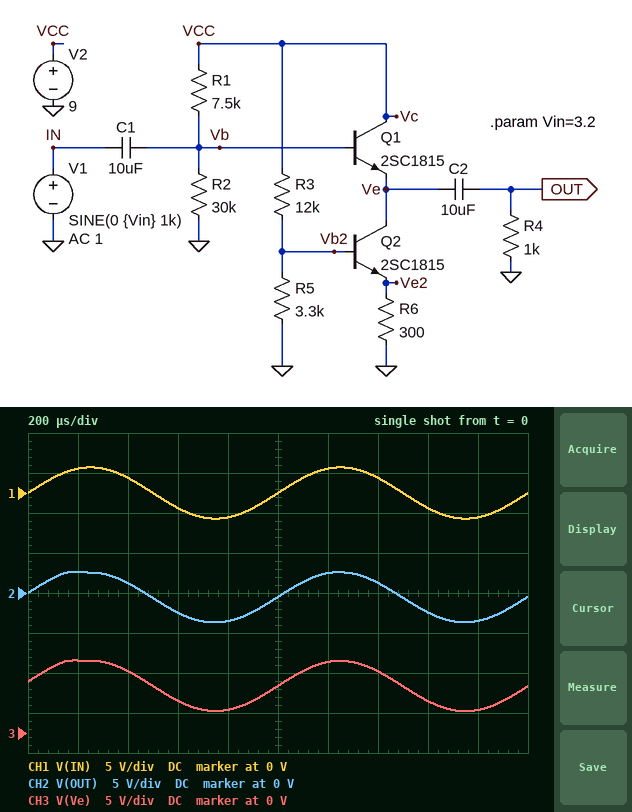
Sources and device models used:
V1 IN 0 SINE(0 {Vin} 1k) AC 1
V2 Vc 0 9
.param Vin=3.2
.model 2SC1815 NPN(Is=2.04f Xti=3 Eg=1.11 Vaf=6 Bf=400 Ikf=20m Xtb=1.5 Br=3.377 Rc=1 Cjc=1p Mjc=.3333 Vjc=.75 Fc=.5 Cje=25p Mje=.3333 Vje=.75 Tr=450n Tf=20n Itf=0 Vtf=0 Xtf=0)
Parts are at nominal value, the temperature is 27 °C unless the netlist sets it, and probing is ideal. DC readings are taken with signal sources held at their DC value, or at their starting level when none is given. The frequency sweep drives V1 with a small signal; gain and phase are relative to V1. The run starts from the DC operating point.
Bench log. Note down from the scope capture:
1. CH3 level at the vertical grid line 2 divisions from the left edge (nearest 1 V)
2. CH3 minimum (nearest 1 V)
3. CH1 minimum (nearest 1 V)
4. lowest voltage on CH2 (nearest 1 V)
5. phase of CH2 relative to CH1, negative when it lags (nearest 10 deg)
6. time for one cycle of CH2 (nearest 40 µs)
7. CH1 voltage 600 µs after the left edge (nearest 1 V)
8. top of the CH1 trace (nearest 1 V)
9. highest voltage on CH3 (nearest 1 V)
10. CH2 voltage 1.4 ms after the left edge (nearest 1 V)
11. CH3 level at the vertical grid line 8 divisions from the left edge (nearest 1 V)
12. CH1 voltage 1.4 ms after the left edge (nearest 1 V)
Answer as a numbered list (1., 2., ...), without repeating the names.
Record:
1. 8 V
2. 3 V
3. -3 V
4. -4 V
5. 0 deg
6. 1.00 ms
7. -2 V
8. 3 V
9. 9 V
10. 1 V
11. 4 V
12. 2 V
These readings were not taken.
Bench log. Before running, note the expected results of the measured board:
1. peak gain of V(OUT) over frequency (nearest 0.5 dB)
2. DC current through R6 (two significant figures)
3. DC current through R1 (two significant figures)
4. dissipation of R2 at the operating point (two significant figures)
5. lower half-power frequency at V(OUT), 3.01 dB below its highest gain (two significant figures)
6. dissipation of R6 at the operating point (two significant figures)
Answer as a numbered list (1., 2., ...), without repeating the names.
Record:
1. 0 dB
2. 4.0 mA
3. 250 µA
4. 1.7 mW
5. 16 Hz
6. 4.8 mW
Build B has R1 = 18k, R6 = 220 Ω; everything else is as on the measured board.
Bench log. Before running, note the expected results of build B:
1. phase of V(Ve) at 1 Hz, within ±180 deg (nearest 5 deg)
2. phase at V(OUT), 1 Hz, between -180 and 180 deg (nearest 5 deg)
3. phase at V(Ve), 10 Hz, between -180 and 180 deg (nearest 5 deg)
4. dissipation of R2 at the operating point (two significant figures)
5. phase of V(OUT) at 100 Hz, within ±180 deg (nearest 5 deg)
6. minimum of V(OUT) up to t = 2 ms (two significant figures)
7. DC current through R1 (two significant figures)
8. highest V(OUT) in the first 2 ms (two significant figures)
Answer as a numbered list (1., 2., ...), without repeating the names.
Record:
1. 55 deg
2. 140 deg
3. 10 deg
4. 1.0 mW
5. 10 deg
6. -3.2 V
7. 190 µA
8. 3.1 V
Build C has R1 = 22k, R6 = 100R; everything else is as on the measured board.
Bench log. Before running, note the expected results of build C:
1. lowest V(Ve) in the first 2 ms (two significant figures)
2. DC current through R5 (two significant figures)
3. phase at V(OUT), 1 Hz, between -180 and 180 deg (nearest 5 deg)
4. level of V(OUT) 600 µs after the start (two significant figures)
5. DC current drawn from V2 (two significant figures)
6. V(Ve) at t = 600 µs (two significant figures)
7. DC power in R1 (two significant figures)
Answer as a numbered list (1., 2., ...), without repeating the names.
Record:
1. 990 mV
2. 570 µA
3. 140 deg
4. -2.0 V
5. 12 mA
6. 2.3 V
7. 760 µW
